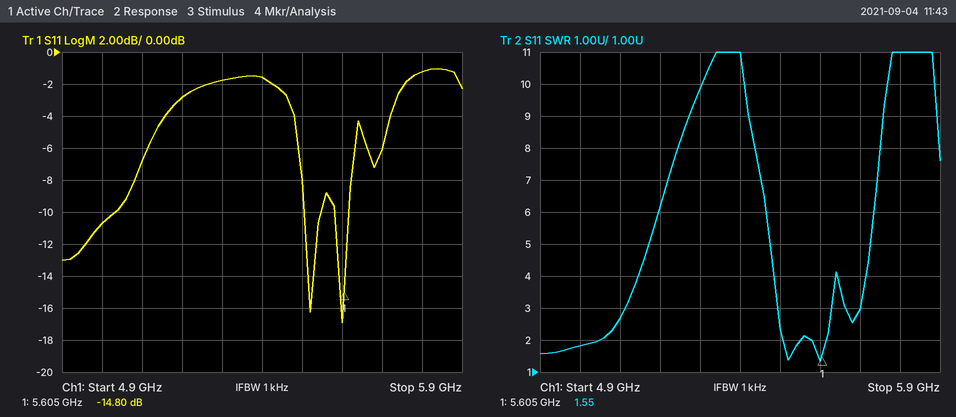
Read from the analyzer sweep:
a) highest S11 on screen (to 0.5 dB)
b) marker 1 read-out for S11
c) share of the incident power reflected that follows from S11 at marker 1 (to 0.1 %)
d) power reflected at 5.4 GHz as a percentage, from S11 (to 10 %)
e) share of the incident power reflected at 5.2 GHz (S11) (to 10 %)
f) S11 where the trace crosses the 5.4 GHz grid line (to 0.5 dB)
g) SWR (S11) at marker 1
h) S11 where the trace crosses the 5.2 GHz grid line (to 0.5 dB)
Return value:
-1.0 dB
-14.80 dB
3.3 %
70 %
50 %
-1.5 dB
1.55
-3.0 dB
